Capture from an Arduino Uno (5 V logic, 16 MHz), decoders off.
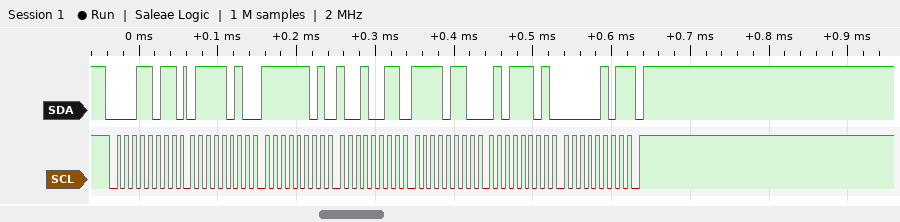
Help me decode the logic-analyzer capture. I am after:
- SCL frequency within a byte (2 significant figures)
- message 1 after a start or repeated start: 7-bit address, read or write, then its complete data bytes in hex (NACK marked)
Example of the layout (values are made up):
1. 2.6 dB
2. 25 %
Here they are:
1. 100 kHz
2. 0x0D read: 7A FD 93 F6 5D 05 NACK
